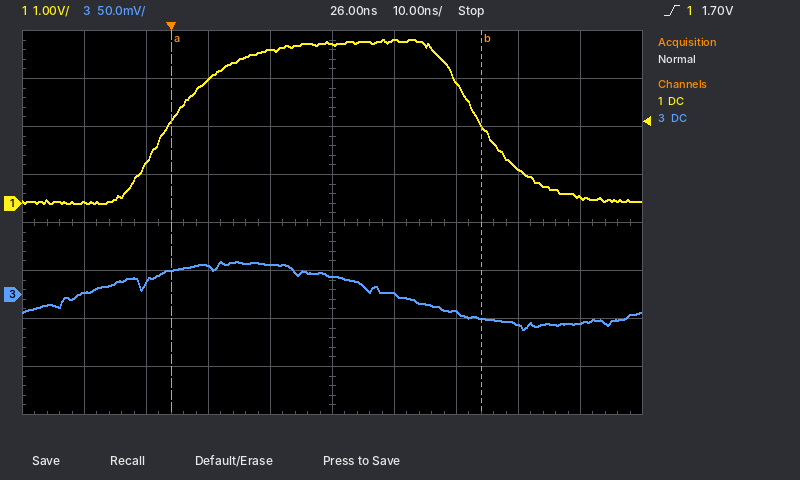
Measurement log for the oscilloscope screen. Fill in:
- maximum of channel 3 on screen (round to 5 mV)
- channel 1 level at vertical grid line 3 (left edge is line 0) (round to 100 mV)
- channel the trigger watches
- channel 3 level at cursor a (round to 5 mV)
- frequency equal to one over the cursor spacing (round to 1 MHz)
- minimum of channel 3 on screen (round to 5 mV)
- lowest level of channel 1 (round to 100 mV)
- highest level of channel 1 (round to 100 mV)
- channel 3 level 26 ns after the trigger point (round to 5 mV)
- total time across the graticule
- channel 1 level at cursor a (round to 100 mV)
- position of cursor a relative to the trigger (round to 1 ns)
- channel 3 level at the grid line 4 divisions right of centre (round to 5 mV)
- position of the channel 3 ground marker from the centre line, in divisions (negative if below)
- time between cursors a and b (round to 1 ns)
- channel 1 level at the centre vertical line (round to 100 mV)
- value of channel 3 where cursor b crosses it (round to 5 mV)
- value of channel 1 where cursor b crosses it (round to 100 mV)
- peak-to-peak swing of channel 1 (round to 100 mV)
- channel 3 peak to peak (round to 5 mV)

35 mV
2.6 V
channel 1
25 mV
20 MHz
-35 mV
0.0 V
3.4 V
20 mV
100 ns
1.7 V
0 ns
-30 mV
-1.5 div
50 ns
3.3 V
-25 mV
1.6 V
3.4 V
70 mV
